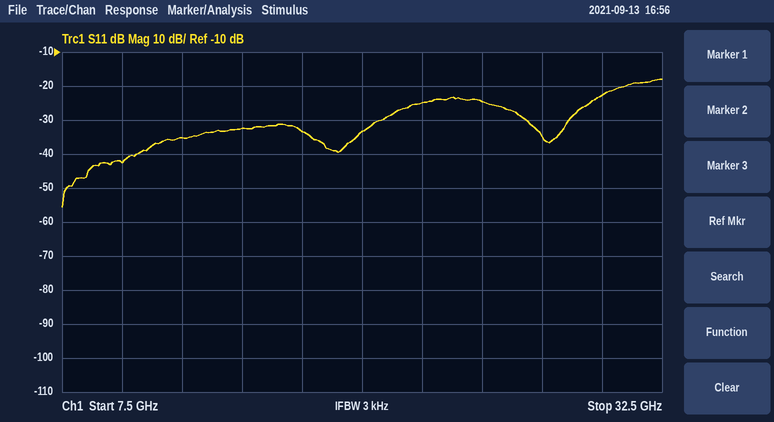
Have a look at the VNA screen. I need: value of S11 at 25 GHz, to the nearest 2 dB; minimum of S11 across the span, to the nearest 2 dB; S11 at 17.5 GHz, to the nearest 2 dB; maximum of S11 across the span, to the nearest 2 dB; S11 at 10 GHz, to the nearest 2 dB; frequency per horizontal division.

-24 dB
-56 dB
-34 dB
-18 dB
-42 dB
2.5 GHz
